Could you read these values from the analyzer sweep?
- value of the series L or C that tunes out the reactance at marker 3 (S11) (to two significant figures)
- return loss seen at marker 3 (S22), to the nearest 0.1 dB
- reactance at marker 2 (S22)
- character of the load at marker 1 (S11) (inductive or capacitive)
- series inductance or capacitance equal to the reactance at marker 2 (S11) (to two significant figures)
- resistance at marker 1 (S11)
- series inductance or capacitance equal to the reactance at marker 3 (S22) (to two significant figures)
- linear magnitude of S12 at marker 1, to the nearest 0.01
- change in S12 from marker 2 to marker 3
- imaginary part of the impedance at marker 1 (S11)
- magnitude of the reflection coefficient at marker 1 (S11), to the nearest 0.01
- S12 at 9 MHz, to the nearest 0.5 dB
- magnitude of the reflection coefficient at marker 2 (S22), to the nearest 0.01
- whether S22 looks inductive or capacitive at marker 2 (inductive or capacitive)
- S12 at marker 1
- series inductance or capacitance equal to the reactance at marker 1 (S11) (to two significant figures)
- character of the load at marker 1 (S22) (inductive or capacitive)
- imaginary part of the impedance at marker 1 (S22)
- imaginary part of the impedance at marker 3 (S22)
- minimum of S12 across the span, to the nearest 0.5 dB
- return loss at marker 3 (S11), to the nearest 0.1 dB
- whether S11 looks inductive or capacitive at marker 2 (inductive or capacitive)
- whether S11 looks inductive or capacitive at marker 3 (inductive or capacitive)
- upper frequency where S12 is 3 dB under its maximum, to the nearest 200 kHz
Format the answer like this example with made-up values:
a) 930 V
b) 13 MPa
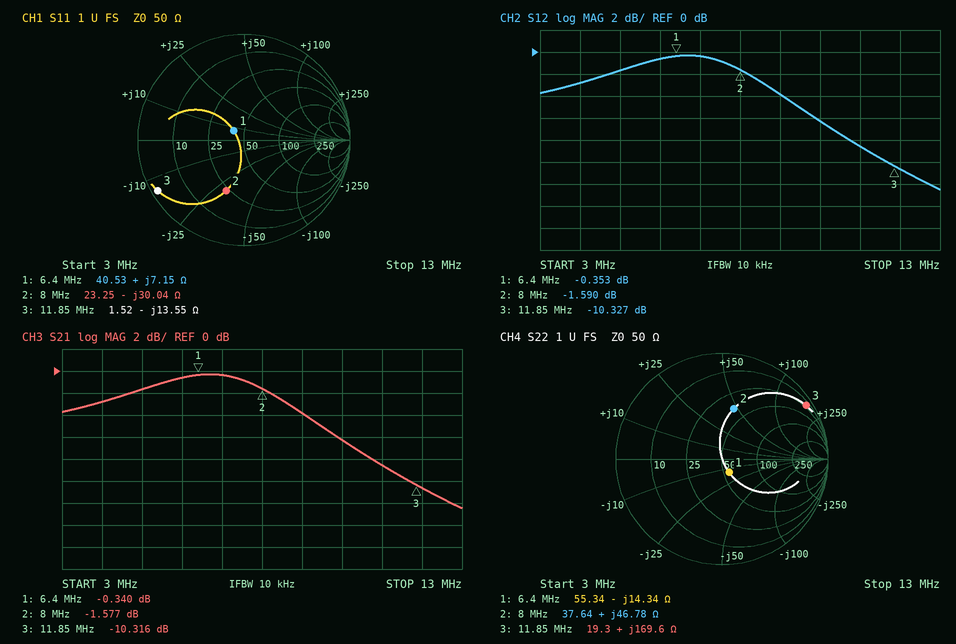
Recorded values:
a) 180 nH
b) 0.5 dB
c) +46.78 Ω
d) inductive
e) 660 pF
f) 40.53 Ω
g) 2.3 µH
h) 0.96
i) -8.737 dB
j) +7.15 Ω
k) 0.13
l) -4.0 dB
m) 0.49
n) inductive
o) -0.353 dB
p) 180 nH
q) capacitive
r) -14.34 Ω
s) +169.6 Ω
t) -12.5 dB
u) 0.5 dB
v) capacitive
w) capacitive
x) 8.8 MHz
